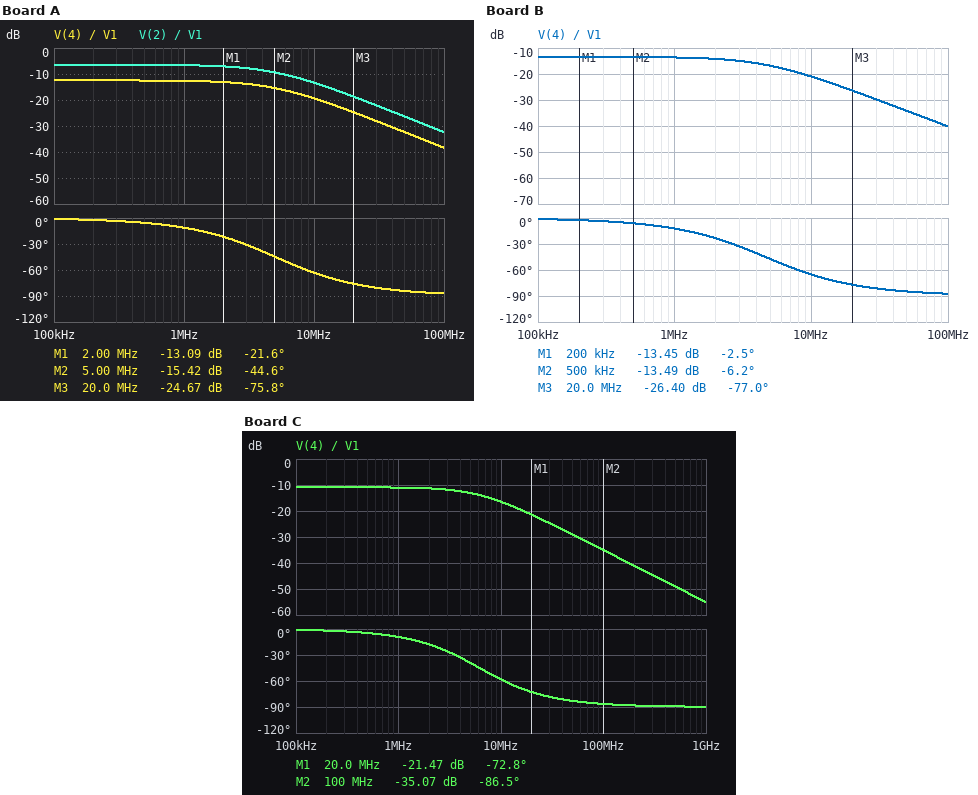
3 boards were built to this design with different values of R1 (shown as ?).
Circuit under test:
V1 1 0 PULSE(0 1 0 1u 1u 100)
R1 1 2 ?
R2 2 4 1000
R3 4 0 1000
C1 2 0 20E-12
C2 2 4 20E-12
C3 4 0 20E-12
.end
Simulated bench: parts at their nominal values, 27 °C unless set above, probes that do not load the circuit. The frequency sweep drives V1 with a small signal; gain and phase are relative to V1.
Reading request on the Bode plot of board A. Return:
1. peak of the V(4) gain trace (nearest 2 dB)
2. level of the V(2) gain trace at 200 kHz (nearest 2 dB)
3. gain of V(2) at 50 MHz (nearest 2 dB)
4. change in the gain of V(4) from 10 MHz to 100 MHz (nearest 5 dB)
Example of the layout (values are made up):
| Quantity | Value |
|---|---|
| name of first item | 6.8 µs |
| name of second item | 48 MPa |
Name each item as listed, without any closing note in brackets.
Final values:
| Quantity | Value |
|---|---|
| peak of the V(4) gain trace | -12 dB |
| level of the V(2) gain trace at 200 kHz | -6 dB |
| gain of V(2) at 50 MHz | -26 dB |
| change in the gain of V(4) from 10 MHz to 100 MHz | -20 dB |
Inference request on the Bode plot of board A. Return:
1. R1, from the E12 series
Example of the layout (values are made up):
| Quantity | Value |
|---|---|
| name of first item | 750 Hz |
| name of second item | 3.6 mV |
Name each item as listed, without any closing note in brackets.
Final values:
| Quantity | Value |
|---|---|
| R1, from the E12 series | 2.2 kΩ |
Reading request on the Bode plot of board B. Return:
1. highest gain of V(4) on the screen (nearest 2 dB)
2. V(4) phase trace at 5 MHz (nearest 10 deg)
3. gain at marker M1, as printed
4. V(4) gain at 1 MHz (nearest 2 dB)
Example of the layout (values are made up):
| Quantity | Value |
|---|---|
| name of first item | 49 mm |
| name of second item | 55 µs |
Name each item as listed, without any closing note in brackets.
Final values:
| Quantity | Value |
|---|---|
| highest gain of V(4) on the screen | -14 dB |
| V(4) phase trace at 5 MHz | -50 deg |
| gain at marker M1, as printed | -13.45 dB |
| V(4) gain at 1 MHz | -14 dB |
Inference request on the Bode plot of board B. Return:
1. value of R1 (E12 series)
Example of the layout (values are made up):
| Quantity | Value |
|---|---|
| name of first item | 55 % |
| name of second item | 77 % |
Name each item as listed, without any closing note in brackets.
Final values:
| Quantity | Value |
|---|---|
| value of R1 | 2.7 kΩ |
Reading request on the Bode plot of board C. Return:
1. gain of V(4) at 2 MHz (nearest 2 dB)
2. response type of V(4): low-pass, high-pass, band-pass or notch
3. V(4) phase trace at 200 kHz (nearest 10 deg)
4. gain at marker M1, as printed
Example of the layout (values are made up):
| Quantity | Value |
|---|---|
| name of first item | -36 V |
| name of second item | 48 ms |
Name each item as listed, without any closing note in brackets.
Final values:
| Quantity | Value |
|---|---|
| gain of V(4) at 2 MHz | -12 dB |
| response type of V(4): low-pass, high-pass, band-pass or notch | low-pass |
| V(4) phase trace at 200 kHz | 0 deg |
| gain at marker M1, as printed | -21.47 dB |
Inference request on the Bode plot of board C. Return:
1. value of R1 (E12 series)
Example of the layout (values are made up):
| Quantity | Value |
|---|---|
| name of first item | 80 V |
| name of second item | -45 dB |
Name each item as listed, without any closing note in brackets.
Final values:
| Quantity | Value |
|---|---|
| value of R1 | 1.5 kΩ |
